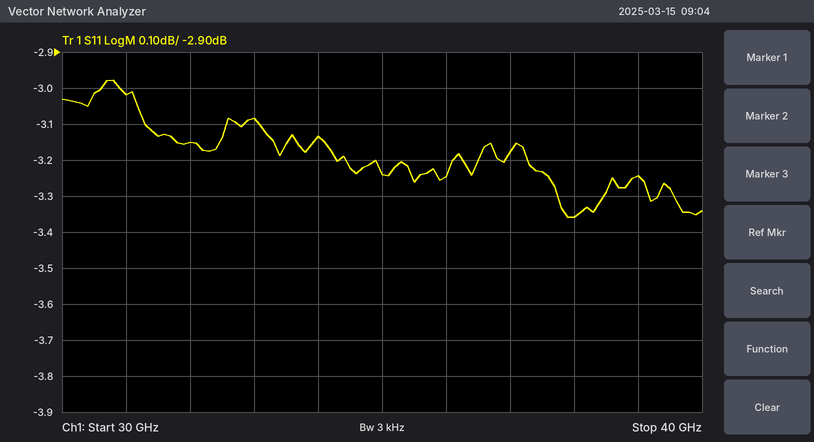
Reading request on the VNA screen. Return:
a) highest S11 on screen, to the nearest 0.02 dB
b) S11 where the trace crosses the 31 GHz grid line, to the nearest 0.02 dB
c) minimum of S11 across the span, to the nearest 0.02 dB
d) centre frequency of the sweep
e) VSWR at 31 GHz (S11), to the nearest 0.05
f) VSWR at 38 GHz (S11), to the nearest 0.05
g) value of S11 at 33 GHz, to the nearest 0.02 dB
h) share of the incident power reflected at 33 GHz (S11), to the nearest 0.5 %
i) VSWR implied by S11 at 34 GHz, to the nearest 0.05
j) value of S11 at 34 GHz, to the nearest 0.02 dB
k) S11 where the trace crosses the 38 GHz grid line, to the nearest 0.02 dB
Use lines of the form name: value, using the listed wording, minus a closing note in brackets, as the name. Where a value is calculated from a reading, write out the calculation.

highest S11 on screen, to the nearest 0.02 dB: -2.98 dB
S11 where the trace crosses the 31 GHz grid line, to the nearest 0.02 dB: -3.02 dB
minimum of S11 across the span, to the nearest 0.02 dB: -3.36 dB
centre frequency of the sweep: 35 GHz
VSWR at 31 GHz (S11), to the nearest 0.05: |Γ| = 10^(-3.02/20) = 0.7063; VSWR = (1 + 0.7063)/(1 − 0.7063) ≈ 5.81, so 5.80 to the nearest 0.05
VSWR at 38 GHz (S11), to the nearest 0.05: |Γ| = 10^(-3.36/20) = 0.6792; VSWR = (1 + 0.6792)/(1 − 0.6792) ≈ 5.23, so 5.25 to the nearest 0.05
value of S11 at 33 GHz, to the nearest 0.02 dB: -3.08 dB
share of the incident power reflected at 33 GHz (S11), to the nearest 0.5 %: 10^(-3.08/10) ≈ 49.2 %, so 49.0 % to the nearest 0.5 %
VSWR implied by S11 at 34 GHz, to the nearest 0.05: |Γ| = 10^(-3.14/20) = 0.6966; VSWR = (1 + 0.6966)/(1 − 0.6966) ≈ 5.59, so 5.60 to the nearest 0.05
value of S11 at 34 GHz, to the nearest 0.02 dB: -3.14 dB
S11 where the trace crosses the 38 GHz grid line, to the nearest 0.02 dB: -3.36 dB
